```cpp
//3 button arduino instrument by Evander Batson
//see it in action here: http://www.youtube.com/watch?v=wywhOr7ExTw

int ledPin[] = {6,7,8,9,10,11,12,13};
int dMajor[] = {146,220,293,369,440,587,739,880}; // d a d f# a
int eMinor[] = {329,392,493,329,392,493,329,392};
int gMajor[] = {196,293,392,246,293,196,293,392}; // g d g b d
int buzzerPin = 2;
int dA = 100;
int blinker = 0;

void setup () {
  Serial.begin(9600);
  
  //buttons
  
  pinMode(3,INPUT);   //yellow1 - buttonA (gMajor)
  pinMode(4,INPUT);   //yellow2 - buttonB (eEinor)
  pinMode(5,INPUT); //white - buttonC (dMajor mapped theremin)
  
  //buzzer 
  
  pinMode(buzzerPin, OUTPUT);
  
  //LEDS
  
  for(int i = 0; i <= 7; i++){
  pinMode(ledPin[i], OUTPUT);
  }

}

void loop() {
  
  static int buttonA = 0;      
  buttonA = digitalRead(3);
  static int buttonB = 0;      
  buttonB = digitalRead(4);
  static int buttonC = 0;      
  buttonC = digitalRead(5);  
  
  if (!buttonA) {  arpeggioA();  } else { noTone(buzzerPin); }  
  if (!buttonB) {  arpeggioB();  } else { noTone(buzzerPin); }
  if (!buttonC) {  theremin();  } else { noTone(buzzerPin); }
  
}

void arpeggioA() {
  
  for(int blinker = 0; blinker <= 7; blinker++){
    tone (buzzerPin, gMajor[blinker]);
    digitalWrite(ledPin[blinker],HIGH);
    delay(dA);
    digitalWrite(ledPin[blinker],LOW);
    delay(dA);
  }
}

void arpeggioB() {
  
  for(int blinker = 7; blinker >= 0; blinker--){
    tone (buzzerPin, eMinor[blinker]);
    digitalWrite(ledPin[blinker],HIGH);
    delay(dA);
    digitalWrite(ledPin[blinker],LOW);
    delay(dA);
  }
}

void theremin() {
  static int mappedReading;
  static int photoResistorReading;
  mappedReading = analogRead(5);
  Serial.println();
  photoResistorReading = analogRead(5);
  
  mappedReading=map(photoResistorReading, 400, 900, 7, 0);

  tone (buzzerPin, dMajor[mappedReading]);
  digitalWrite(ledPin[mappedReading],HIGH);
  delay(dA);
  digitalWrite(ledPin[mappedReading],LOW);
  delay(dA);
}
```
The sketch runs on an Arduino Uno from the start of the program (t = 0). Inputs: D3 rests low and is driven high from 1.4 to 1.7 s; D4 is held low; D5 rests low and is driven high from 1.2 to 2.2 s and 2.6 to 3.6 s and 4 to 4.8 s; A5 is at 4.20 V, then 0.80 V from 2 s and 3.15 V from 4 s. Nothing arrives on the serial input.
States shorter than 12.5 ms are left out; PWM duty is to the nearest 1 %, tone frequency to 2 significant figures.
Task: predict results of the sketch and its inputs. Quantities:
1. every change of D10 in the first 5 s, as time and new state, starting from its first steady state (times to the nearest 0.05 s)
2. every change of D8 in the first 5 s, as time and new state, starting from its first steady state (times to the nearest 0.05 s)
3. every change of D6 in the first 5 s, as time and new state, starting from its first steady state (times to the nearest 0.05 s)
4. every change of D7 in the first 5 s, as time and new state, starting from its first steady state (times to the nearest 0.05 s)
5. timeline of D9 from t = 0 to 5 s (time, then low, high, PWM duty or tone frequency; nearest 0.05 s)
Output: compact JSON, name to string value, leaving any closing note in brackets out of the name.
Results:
{"every change of D10 in the first 5 s, as time and new state, starting from its first steady state": "0 s low; 0.8 s high; 0.9 s low; 2.2 s high; 2.3 s low; 4.2 s high; 4.3 s low", "every change of D8 in the first 5 s, as time and new state, starting from its first steady state": "0 s low; 0.4 s high; 0.5 s low; 2.6 s high; 2.7 s low; 3.8 s high; 3.9 s low", "every change of D6 in the first 5 s, as time and new state, starting from its first steady state": "0 s high; 0.1 s low; 3 s high; 3.1 s low; 3.4 s high; 3.5 s low", "every change of D7 in the first 5 s, as time and new state, starting from its first steady state": "0 s low; 0.2 s high; 0.3 s low; 2.8 s high; 2.9 s low; 3.6 s high; 3.7 s low", "timeline of D9 from t = 0 to 5 s": "0 s low; 0.6 s high; 0.7 s low; 2.4 s high; 2.5 s low; 4 s high; 4.1 s low"}
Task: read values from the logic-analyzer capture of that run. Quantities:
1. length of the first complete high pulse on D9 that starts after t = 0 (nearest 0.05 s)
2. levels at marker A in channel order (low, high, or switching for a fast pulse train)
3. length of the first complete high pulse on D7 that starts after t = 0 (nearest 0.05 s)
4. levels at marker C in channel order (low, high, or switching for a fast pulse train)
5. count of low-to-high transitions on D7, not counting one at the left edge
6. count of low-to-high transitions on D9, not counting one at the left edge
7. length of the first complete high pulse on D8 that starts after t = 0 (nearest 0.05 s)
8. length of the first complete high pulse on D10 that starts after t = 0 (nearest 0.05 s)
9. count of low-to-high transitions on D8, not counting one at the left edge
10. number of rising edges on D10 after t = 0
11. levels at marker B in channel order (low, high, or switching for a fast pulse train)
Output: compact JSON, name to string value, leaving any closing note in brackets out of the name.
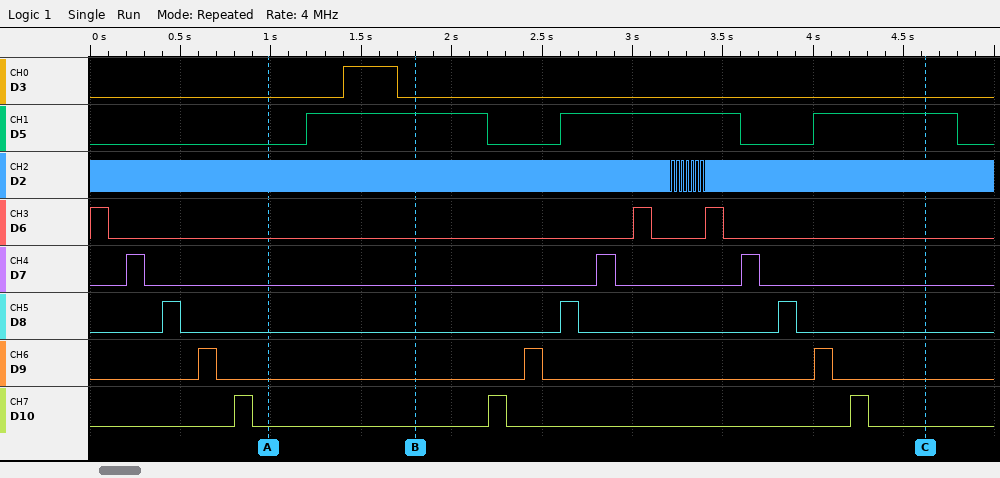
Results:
{"length of the first complete high pulse on D9 that starts after t = 0": "0.10 s", "levels at marker A in channel order": "D3 low, D5 low, D2 switching, D6 low, D7 low, D8 low, D9 low, D10 low", "length of the first complete high pulse on D7 that starts after t = 0": "0.10 s", "levels at marker C in channel order": "D3 low, D5 high, D2 switching, D6 low, D7 low, D8 low, D9 low, D10 low", "count of low-to-high transitions on D7, not counting one at the left edge": "3", "count of low-to-high transitions on D9, not counting one at the left edge": "3", "length of the first complete high pulse on D8 that starts after t = 0": "0.10 s", "length of the first complete high pulse on D10 that starts after t = 0": "0.10 s", "count of low-to-high transitions on D8, not counting one at the left edge": "3", "number of rising edges on D10 after t = 0": "3", "levels at marker B in channel order": "D3 low, D5 high, D2 switching, D6 low, D7 low, D8 low, D9 low, D10 low"}
